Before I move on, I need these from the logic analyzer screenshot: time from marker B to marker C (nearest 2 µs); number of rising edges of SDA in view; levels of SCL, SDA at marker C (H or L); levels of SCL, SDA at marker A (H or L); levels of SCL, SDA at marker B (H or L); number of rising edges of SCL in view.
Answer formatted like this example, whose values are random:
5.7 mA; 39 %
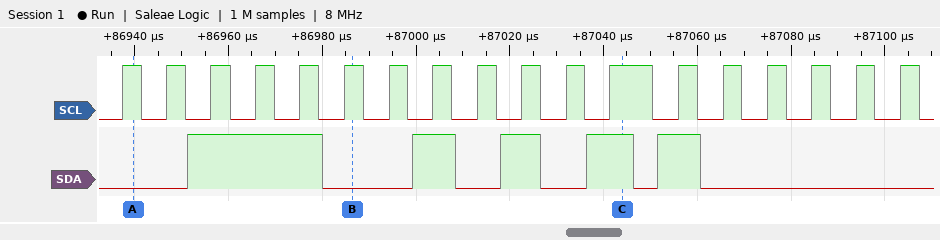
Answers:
58 µs; 5; SCL=H, SDA=H; SCL=H, SDA=L; SCL=H, SDA=L; 18
